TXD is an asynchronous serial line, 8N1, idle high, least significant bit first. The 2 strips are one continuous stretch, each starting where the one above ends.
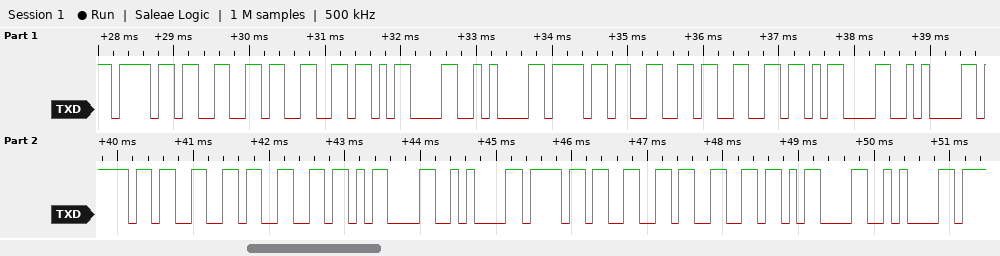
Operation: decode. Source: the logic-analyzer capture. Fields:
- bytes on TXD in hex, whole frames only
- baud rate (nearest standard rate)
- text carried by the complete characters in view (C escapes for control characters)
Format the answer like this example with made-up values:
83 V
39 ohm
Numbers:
6F 66 66 0D 0A 6F 66 66 0D 0A 6F 66 66 0D 0A 6F 66 66 0D 0A
9600 baud
"off\r\noff\r\noff\r\noff\r\n"
